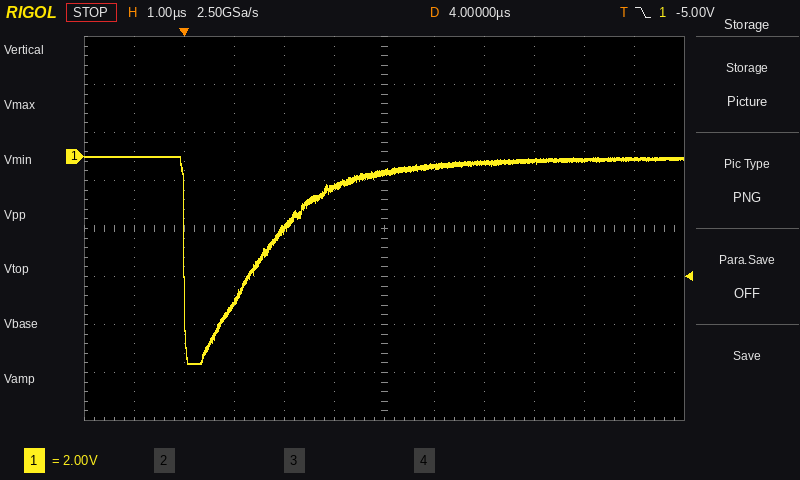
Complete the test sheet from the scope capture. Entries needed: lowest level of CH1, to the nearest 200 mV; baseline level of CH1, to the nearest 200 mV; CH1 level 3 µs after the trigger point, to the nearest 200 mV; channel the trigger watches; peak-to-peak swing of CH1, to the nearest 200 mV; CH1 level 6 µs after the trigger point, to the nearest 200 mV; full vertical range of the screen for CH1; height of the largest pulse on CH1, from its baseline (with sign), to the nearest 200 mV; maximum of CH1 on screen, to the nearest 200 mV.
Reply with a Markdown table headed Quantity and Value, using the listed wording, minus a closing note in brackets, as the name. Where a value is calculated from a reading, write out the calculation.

| Quantity | Value |
|---|---|
| lowest level of CH1, to the nearest 200 mV | -8.6 V |
| baseline level of CH1, to the nearest 200 mV | -200 mV |
| CH1 level 3 µs after the trigger point, to the nearest 200 mV | -1.2 V |
| channel the trigger watches | CH1 |
| peak-to-peak swing of CH1, to the nearest 200 mV | 0.0 V − (-8.6 V) = 8.6 V |
| CH1 level 6 µs after the trigger point, to the nearest 200 mV | -200 mV |
| full vertical range of the screen for CH1 | 16 V |
| height of the largest pulse on CH1, from its baseline (with sign), to the nearest 200 mV | -8.6 V − (-200 mV) = -8.4 V |
| maximum of CH1 on screen, to the nearest 200 mV | 0.0 V |
